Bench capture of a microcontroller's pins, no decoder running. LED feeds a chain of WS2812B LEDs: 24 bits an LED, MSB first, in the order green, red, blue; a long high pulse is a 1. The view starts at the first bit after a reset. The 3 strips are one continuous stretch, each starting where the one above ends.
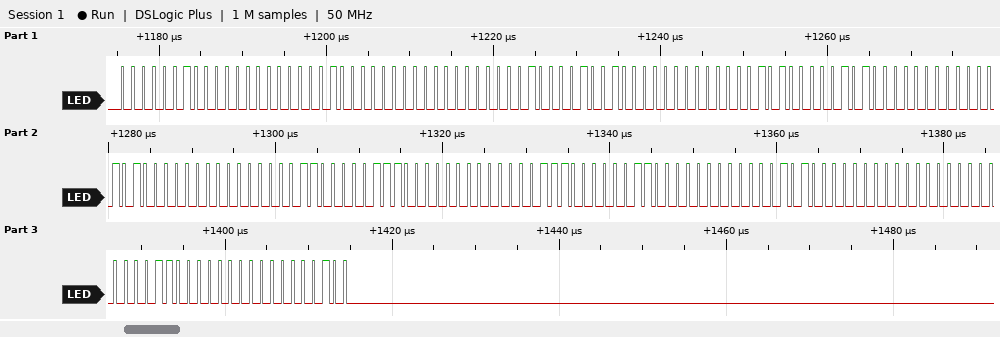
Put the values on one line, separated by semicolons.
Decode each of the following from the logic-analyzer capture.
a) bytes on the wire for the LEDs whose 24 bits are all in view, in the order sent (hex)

02 00 08 00 01 09 00 05 05 00 0A 00 03 07 00 07 03 00 0A 00 00 06 00 04
